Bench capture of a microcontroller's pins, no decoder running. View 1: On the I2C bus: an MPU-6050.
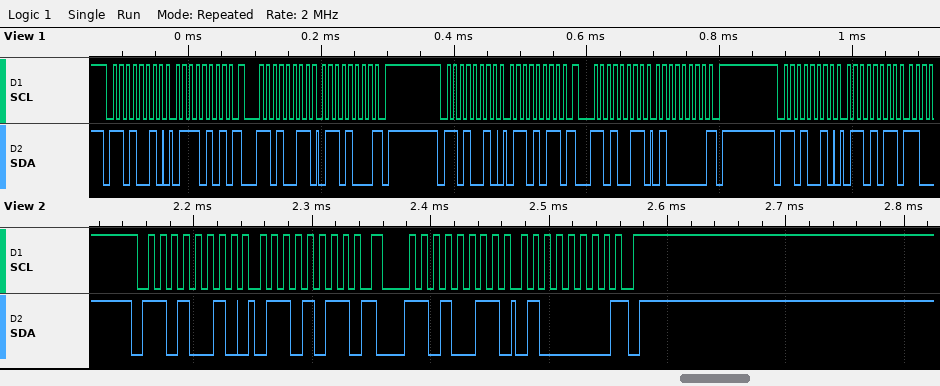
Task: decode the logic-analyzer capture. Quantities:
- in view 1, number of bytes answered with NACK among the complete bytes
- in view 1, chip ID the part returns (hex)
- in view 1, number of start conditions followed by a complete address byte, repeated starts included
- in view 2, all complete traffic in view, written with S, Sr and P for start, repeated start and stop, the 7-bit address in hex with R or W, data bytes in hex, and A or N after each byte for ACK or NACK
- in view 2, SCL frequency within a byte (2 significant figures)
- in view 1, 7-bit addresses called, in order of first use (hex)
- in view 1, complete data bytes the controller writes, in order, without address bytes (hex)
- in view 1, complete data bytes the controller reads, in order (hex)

2
0x68
5
S 69W A 6B A Sr 69R A 40 N P
100 kHz
0x69
75 6B 6B
68 40
